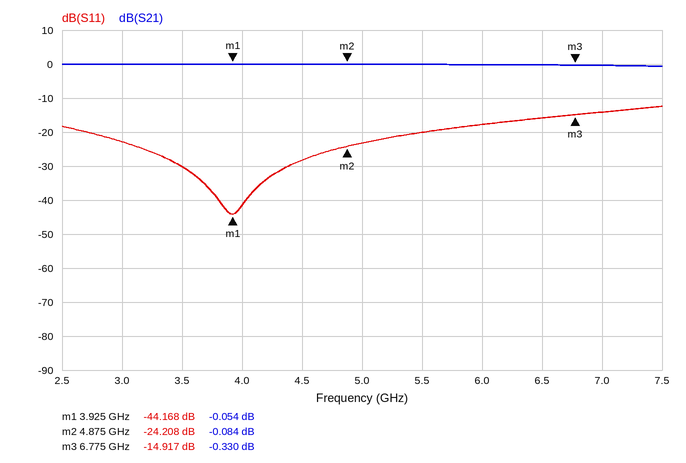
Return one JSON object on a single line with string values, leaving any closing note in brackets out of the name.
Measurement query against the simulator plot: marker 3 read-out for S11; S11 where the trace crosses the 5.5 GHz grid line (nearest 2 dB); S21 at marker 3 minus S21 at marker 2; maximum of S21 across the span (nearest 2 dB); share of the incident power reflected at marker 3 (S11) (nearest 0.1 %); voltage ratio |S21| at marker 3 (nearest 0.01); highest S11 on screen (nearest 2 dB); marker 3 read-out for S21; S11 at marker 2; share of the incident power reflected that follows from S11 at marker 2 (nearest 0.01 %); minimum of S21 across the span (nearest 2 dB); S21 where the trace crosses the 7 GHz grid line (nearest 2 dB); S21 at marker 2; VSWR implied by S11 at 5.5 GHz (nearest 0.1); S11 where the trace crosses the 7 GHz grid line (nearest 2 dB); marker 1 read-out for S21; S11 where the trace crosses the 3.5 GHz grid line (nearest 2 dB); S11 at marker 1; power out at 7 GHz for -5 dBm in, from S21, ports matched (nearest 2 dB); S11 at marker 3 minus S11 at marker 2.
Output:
{"marker 3 read-out for S11": "-14.917 dB", "S11 where the trace crosses the 5.5 GHz grid line": "-20 dB", "S21 at marker 3 minus S21 at marker 2": "-0.246 dB", "maximum of S21 across the span": "0 dB", "share of the incident power reflected at marker 3 (S11)": "3.2 %", "voltage ratio |S21| at marker 3": "0.96", "highest S11 on screen": "-12 dB", "marker 3 read-out for S21": "-0.330 dB", "S11 at marker 2": "-24.208 dB", "share of the incident power reflected that follows from S11 at marker 2": "0.38 %", "minimum of S21 across the span": "0 dB", "S21 where the trace crosses the 7 GHz grid line": "0 dB", "S21 at marker 2": "-0.084 dB", "VSWR implied by S11 at 5.5 GHz": "1.2", "S11 where the trace crosses the 7 GHz grid line": "-14 dB", "marker 1 read-out for S21": "-0.054 dB", "S11 where the trace crosses the 3.5 GHz grid line": "-30 dB", "S11 at marker 1": "-44.168 dB", "power out at 7 GHz for -5 dBm in, from S21, ports matched": "-6 dBm", "S11 at marker 3 minus S11 at marker 2": "9.291 dB"}
